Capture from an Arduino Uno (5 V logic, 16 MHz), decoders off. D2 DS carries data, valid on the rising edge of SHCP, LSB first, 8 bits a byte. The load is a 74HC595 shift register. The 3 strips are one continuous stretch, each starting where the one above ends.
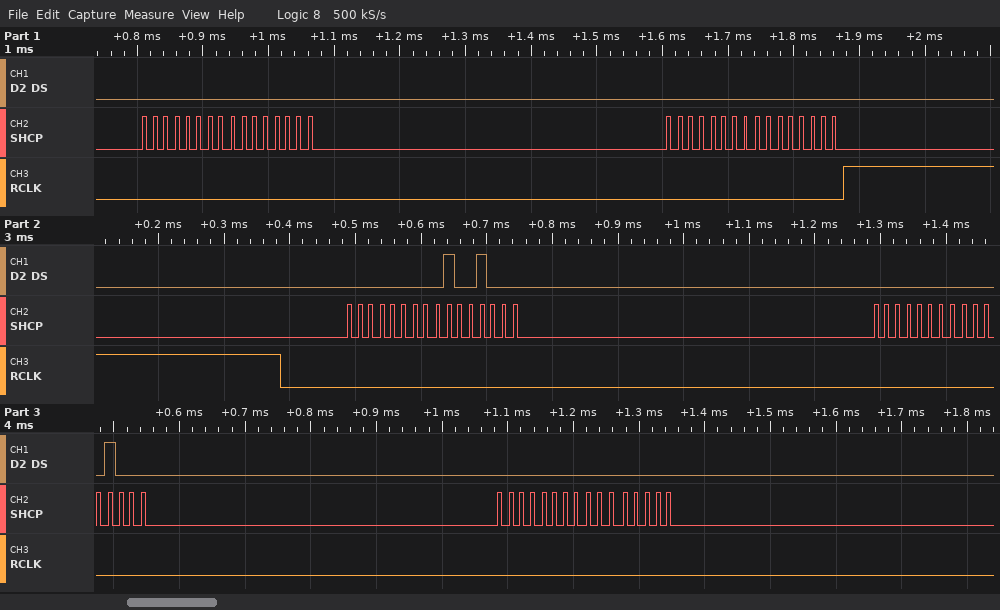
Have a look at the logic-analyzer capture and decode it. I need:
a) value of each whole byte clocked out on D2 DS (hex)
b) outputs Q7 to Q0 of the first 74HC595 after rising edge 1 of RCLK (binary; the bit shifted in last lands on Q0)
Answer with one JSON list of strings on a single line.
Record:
["00 00 00 00 00 12 00 10 00 00", "00000000"]
